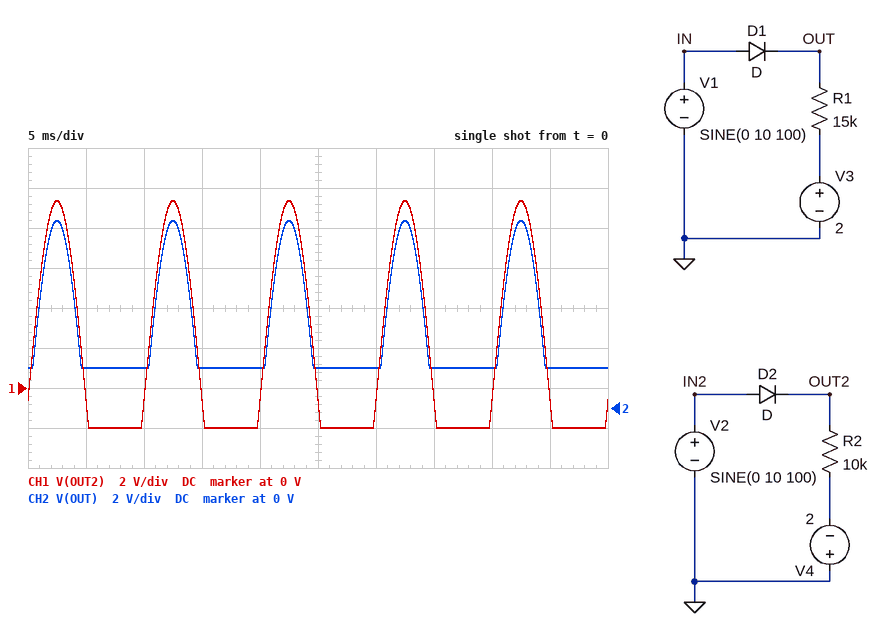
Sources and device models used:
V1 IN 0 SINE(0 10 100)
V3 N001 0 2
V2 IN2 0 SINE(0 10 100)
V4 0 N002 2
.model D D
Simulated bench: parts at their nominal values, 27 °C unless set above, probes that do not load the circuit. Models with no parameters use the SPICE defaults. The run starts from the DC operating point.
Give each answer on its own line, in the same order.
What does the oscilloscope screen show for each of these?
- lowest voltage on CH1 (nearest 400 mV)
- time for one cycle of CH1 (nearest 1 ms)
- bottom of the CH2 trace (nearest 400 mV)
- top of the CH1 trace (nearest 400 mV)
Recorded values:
-2.0 V
10 ms
2.0 V
9.2 V
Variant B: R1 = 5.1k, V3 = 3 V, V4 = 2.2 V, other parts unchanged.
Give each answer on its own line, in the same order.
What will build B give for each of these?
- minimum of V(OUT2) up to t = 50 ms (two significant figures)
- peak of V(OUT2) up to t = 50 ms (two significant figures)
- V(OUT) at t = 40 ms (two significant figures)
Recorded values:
-2.2 V
9.3 V
3.0 V
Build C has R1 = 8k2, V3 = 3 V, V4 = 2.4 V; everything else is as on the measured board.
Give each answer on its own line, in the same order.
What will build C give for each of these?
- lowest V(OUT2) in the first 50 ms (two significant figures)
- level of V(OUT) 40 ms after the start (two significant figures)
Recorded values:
-2.4 V
3.0 V
